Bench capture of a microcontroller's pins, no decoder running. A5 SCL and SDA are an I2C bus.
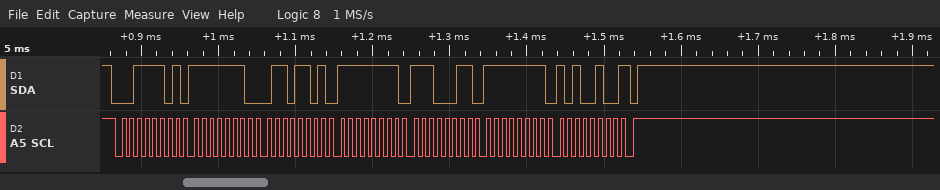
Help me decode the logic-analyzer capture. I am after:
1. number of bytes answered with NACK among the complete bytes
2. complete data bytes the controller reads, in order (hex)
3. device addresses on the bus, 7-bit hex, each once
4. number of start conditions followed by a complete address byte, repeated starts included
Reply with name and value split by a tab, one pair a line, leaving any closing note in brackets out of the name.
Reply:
number of bytes answered with NACK among the complete bytes	1
complete data bytes the controller reads, in order	FE 6D FF E3 FF A4
device addresses on the bus, 7-bit hex, each once	0x1E
number of start conditions followed by a complete address byte, repeated starts included	1
